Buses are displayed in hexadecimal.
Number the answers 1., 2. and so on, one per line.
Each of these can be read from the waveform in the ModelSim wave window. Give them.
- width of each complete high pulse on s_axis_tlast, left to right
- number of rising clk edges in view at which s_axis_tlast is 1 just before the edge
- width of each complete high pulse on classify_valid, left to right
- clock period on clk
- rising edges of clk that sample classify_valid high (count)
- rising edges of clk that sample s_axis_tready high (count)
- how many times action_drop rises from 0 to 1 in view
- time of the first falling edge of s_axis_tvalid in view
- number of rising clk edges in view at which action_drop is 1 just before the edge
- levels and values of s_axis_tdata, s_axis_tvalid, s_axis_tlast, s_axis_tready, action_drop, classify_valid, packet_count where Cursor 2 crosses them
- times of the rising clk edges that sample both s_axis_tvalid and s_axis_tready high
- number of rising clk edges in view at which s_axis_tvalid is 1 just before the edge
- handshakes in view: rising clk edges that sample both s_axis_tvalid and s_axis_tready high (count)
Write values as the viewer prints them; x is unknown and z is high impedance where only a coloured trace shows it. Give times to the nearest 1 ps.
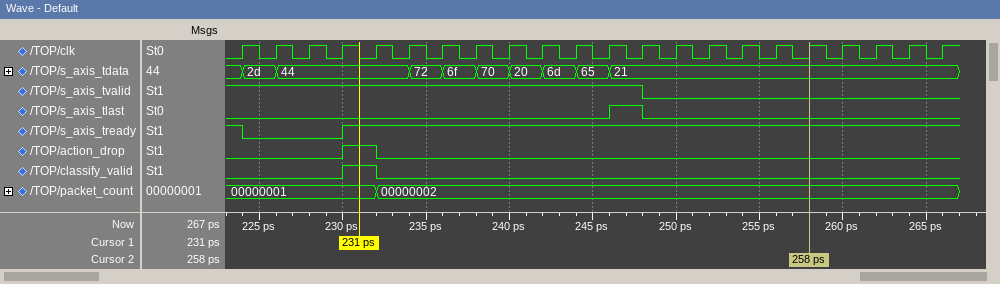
1. 2 ps
2. 1
3. 2 ps
4. 2 ps
5. 1
6. 19
7. 1
8. 248 ps
9. 1
10. s_axis_tdata=21, s_axis_tvalid=0, s_axis_tlast=0, s_axis_tready=1, action_drop=0, classify_valid=0, packet_count=00000002
11. 224 ps, 232 ps, 234 ps, 236 ps, 238 ps, 240 ps, 242 ps, 244 ps, 246 ps, 248 ps
12. 13
13. 10
